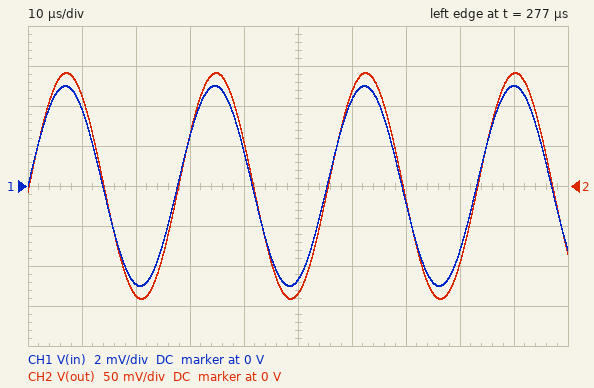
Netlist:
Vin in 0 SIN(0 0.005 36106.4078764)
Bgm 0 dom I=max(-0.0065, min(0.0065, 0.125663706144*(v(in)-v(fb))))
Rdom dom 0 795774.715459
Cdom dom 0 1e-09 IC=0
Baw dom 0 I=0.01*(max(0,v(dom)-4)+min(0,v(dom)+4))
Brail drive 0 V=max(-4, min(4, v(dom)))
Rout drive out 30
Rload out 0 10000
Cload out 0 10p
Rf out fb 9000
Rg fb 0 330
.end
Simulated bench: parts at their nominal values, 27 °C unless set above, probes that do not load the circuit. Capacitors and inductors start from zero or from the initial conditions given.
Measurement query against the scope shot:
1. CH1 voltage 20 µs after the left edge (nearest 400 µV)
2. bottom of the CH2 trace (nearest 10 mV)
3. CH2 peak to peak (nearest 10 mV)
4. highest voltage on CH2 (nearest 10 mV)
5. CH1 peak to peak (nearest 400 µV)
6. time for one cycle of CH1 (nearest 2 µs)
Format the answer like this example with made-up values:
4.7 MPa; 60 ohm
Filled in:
-4.8 mV; -140 mV; 280 mV; 140 mV; 10.0 mV; 28 µs
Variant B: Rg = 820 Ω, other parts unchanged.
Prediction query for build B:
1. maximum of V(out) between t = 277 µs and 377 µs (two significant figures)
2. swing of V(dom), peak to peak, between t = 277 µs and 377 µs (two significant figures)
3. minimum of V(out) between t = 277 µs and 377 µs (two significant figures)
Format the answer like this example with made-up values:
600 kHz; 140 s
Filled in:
60 mV; 120 mV; -60 mV
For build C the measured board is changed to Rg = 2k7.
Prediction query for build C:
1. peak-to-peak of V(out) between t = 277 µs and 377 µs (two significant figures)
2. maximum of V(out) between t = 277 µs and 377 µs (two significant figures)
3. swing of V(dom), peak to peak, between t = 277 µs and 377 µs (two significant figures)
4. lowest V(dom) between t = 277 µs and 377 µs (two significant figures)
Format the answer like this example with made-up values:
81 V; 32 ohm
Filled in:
43 mV; 22 mV; 44 mV; -22 mV
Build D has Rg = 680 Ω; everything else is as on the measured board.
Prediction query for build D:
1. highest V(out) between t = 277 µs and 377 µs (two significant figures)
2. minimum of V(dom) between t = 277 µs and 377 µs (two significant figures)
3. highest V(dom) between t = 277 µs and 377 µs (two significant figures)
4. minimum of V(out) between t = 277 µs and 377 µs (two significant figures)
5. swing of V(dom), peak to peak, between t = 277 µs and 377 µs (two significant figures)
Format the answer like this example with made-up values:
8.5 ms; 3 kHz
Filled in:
71 mV; -72 mV; 72 mV; -71 mV; 140 mV
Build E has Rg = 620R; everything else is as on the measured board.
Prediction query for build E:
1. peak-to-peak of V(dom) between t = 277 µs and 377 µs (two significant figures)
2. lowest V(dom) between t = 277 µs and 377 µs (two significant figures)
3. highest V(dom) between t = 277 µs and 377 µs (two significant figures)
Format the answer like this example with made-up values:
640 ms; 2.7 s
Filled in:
160 mV; -78 mV; 78 mV
